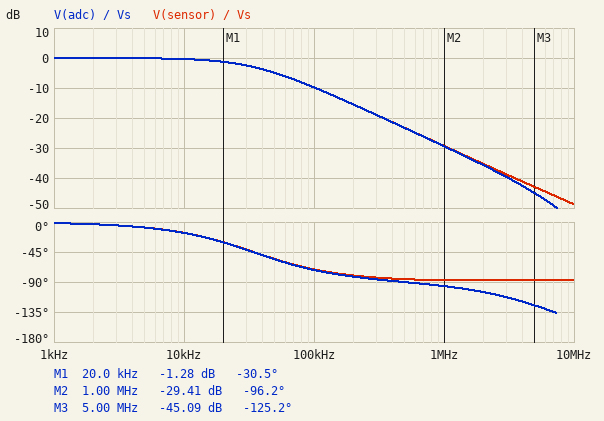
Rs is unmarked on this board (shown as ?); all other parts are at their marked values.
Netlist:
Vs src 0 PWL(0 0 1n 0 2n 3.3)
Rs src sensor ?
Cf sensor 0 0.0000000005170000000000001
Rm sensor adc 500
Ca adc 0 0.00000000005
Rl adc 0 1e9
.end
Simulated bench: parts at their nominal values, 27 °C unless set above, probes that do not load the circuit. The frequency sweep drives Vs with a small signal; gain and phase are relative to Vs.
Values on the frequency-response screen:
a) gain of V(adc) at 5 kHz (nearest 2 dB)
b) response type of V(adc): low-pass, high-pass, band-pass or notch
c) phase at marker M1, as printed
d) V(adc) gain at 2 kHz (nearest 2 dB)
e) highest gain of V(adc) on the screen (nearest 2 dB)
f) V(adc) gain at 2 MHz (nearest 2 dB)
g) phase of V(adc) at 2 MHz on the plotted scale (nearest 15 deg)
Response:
0 dB
low-pass
-30.5 deg
0 dB
0 dB
-36 dB
-105 deg
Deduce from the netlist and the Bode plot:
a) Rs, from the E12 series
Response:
8.2 kΩ
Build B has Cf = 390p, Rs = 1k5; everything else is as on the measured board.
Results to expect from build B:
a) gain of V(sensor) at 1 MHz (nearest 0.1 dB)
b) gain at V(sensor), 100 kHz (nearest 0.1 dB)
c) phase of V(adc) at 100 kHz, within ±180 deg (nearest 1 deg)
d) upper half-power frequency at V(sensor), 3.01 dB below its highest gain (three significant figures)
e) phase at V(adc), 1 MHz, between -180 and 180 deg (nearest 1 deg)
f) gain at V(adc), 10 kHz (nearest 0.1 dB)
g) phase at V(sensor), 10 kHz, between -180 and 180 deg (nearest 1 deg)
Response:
-12.6 dB
-0.7 dB
-23 deg
240 kHz
-84 deg
0 dB
-2 deg
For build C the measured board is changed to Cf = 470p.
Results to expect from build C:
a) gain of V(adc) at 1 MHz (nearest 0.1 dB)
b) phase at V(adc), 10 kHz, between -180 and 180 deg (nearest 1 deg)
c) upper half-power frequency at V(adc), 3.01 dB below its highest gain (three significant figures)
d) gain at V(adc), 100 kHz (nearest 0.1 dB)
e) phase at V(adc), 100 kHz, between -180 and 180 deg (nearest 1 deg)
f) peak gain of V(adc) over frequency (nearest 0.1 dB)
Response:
-28.7 dB
-15 deg
37.3 kHz
-9.1 dB
-70 deg
0 dB
